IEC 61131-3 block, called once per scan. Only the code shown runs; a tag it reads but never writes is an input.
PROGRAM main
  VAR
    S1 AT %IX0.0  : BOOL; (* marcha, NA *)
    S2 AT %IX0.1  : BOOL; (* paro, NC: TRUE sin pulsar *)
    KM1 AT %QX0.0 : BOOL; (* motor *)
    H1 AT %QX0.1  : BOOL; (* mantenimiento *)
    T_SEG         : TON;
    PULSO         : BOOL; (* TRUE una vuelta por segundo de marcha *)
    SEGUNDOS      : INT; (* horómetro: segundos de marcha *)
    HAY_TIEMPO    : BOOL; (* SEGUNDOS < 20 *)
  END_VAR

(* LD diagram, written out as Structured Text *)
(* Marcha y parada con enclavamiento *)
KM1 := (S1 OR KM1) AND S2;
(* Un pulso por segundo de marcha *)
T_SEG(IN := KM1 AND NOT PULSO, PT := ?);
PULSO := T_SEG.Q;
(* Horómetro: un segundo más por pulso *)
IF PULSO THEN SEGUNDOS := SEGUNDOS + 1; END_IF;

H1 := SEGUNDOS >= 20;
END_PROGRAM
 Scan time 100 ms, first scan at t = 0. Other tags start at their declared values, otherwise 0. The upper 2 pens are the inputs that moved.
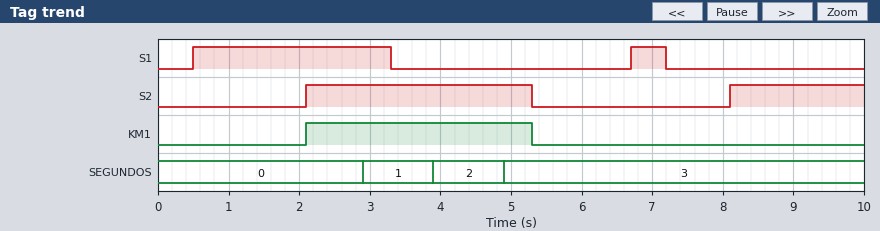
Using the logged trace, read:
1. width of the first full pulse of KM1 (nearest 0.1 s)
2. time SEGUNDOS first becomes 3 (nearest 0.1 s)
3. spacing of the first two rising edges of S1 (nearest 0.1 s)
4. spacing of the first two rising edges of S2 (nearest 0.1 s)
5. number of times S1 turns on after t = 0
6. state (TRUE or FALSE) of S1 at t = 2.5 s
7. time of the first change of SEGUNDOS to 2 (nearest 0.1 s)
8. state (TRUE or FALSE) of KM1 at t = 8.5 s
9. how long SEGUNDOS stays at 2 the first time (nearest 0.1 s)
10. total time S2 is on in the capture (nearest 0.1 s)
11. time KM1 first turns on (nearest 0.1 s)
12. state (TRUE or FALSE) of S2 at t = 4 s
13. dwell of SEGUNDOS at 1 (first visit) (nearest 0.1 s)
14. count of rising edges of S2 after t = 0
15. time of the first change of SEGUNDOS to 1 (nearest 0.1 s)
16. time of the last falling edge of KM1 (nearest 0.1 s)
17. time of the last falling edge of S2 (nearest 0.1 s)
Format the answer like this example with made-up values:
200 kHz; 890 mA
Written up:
3.2 s; 4.9 s; 6.2 s; 6.0 s; 2; TRUE; 3.9 s; FALSE; 1.0 s; 5.1 s; 2.1 s; TRUE; 1.0 s; 2; 2.9 s; 5.3 s; 5.3 s
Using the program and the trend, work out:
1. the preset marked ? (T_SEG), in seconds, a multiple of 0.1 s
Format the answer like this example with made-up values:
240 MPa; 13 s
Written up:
0.8 s
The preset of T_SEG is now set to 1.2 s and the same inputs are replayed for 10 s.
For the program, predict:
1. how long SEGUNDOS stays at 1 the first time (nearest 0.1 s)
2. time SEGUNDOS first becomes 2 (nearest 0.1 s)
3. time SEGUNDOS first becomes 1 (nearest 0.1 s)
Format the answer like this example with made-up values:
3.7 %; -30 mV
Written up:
1.4 s; 4.7 s; 3.3 s
